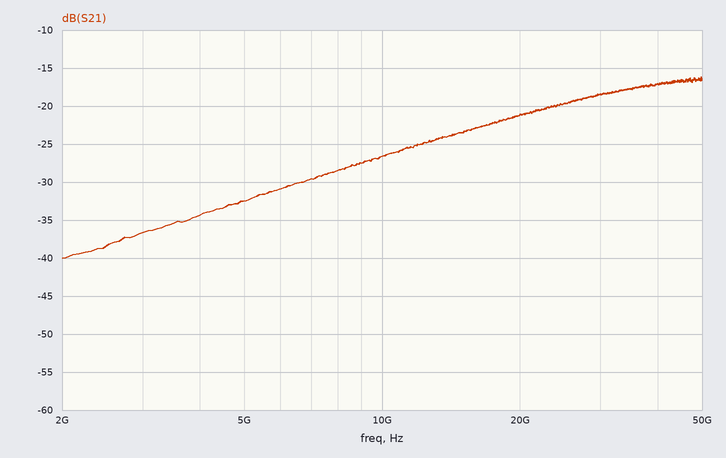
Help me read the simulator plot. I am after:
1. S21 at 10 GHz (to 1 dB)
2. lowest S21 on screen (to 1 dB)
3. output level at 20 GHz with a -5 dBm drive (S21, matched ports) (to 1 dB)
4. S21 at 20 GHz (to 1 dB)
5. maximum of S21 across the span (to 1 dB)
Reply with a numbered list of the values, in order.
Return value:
1. -27 dB
2. -40 dB
3. -26 dBm
4. -21 dB
5. -16 dB
